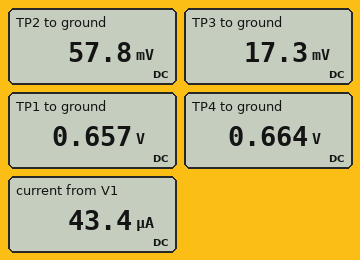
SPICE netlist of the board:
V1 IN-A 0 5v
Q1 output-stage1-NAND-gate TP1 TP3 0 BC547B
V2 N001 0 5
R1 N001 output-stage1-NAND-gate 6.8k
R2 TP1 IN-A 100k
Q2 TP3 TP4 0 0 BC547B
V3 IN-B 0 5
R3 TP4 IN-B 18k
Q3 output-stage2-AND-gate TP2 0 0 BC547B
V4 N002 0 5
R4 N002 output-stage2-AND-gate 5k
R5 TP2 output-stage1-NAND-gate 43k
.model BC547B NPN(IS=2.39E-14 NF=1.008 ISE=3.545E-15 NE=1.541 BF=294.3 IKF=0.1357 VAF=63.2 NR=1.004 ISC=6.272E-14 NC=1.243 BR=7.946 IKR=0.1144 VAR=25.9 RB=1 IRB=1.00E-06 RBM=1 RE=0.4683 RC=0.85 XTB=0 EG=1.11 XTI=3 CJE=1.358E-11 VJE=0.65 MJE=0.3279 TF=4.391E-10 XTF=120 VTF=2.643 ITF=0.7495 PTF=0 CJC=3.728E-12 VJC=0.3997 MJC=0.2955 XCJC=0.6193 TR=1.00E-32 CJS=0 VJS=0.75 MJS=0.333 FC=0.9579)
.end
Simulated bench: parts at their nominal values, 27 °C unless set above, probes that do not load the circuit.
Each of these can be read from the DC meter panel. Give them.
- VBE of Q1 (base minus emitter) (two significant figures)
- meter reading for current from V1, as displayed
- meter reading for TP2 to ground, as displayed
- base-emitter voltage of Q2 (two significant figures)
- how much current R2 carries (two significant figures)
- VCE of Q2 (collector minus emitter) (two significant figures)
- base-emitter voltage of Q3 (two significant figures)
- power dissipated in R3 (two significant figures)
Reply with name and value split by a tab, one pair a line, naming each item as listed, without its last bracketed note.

VBE of Q1 (base minus emitter)	640 mV
meter reading for current from V1, as displayed	43.4 µA
meter reading for TP2 to ground, as displayed	57.8 mV
base-emitter voltage of Q2	660 mV
how much current R2 carries	43 µA
VCE of Q2 (collector minus emitter)	17 mV
base-emitter voltage of Q3	58 mV
power dissipated in R3	1.0 mW
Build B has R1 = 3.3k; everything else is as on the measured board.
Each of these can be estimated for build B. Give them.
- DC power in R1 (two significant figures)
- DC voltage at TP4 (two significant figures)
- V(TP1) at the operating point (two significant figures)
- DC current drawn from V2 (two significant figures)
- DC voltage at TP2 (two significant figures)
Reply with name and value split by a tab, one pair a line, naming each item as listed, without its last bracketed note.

DC power in R1	7.3 mW
DC voltage at TP4	670 mV
V(TP1) at the operating point	680 mV
DC current drawn from V2	1.5 mA
DC voltage at TP2	84 mV
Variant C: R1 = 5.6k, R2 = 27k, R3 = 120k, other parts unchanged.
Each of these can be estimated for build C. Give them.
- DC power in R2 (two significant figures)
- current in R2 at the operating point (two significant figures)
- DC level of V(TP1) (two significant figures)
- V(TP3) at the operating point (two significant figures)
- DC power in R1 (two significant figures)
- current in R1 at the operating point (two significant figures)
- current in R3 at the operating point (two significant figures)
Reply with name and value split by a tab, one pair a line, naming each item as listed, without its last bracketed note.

DC power in R2	680 µW
current in R2 at the operating point	160 µA
DC level of V(TP1)	710 mV
V(TP3) at the operating point	53 mV
DC power in R1	4.3 mW
current in R1 at the operating point	880 µA
current in R3 at the operating point	36 µA
